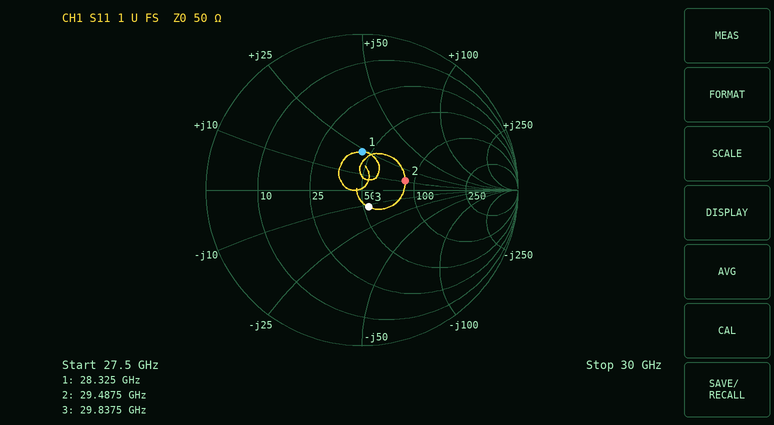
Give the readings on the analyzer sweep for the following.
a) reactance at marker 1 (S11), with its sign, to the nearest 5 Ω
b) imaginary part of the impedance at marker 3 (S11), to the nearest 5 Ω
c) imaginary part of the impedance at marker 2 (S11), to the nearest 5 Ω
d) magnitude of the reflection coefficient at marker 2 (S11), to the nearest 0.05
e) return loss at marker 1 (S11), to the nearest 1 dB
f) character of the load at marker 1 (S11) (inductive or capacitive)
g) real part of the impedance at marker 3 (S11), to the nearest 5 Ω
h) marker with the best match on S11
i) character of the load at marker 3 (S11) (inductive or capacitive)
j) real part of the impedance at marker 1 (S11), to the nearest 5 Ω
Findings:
+25 Ω
-10 Ω
+10 Ω
0.30
12 dB
inductive
55 Ω
marker 3
capacitive
45 Ω
